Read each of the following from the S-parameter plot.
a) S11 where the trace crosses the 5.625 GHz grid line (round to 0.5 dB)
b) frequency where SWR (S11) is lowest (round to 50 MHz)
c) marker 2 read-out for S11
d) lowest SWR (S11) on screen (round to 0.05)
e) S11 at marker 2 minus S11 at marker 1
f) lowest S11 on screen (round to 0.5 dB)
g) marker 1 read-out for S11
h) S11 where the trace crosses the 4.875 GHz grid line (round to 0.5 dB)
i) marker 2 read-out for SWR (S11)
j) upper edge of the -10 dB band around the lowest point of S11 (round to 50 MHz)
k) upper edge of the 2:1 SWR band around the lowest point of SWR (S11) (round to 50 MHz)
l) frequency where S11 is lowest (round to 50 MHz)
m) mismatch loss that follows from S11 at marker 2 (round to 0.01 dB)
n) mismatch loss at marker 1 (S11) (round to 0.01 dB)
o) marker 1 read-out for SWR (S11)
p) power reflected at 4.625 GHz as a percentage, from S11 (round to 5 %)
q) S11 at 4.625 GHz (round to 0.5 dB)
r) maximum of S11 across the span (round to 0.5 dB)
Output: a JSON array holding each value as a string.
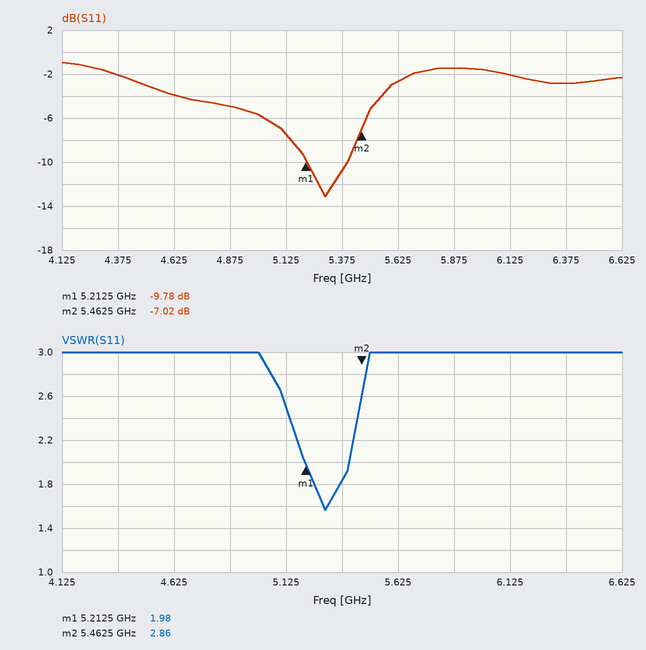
["-2.5 dB", "5.30 GHz", "-7.02 dB", "1.55", "2.76 dB", "-13.0 dB", "-9.78 dB", "-5.0 dB", "2.86", "5.40 GHz", "5.40 GHz", "5.30 GHz", "0.96 dB", "0.48 dB", "1.98", "40 %", "-4.0 dB", "-1.0 dB"]
